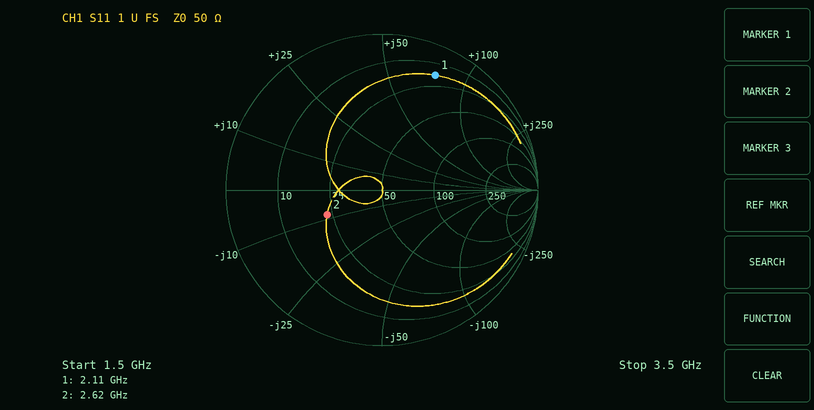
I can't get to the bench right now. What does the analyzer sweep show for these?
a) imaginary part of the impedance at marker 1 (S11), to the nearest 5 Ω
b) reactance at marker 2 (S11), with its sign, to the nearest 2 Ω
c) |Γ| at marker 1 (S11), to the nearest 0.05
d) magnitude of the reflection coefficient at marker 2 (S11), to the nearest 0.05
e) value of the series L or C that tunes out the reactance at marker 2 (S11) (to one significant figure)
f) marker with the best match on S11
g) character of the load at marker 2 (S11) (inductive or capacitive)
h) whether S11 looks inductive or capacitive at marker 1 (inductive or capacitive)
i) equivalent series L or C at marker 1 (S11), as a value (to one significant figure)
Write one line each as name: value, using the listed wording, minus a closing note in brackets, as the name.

imaginary part of the impedance at marker 1 (S11), to the nearest 5 Ω: +75 Ω
reactance at marker 2 (S11), with its sign, to the nearest 2 Ω: -8 Ω
|Γ| at marker 1 (S11), to the nearest 0.05: 0.80
magnitude of the reflection coefficient at marker 2 (S11), to the nearest 0.05: 0.40
value of the series L or C that tunes out the reactance at marker 2 (S11): 500 pH
marker with the best match on S11: marker 2
character of the load at marker 2 (S11): capacitive
whether S11 looks inductive or capacitive at marker 1: inductive
equivalent series L or C at marker 1 (S11), as a value: 6 nH
